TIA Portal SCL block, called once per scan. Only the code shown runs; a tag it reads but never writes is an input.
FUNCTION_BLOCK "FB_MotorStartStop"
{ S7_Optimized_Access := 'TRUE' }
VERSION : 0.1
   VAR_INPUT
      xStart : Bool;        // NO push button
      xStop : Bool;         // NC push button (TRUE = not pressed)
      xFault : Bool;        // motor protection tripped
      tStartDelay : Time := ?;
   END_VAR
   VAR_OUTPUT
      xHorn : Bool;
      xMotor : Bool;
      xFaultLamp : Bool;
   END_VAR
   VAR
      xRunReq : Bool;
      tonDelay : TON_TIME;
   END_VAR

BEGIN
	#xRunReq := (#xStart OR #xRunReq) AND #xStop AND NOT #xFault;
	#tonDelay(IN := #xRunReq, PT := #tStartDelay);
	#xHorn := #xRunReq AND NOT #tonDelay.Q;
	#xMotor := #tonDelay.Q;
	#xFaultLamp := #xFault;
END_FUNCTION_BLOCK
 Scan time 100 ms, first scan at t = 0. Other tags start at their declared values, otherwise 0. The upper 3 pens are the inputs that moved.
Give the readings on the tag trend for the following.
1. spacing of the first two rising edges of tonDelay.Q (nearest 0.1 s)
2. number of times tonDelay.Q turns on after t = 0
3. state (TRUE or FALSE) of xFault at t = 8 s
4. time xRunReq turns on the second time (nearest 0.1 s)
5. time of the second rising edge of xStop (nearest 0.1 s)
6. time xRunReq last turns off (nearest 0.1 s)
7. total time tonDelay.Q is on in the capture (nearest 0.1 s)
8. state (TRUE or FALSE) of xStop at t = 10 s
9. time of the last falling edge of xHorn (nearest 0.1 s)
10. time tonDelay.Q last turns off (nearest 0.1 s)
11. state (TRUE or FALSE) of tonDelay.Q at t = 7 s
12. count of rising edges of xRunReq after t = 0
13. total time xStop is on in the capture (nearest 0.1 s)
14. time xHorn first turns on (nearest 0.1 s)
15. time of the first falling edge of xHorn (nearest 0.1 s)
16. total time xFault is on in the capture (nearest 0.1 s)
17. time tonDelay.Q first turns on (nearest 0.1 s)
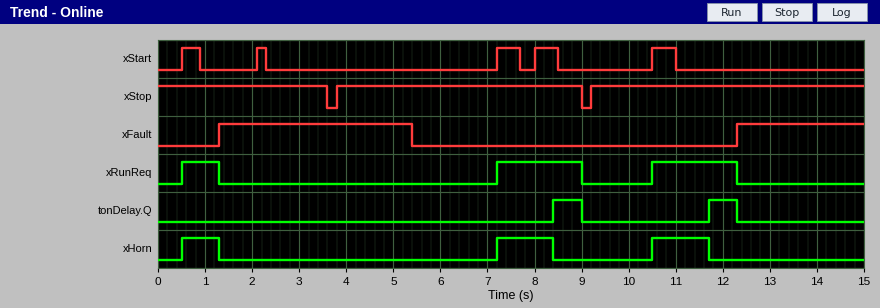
3.3 s
2
FALSE
7.2 s
9.2 s
12.3 s
1.2 s
TRUE
11.7 s
12.3 s
FALSE
3
14.6 s
0.5 s
1.3 s
6.8 s
8.4 s
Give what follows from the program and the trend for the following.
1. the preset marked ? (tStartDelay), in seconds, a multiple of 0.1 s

1.2 s
